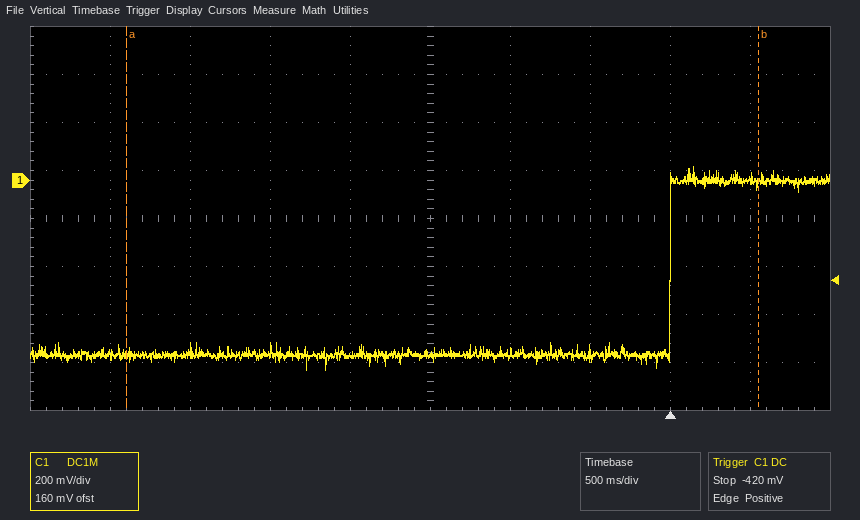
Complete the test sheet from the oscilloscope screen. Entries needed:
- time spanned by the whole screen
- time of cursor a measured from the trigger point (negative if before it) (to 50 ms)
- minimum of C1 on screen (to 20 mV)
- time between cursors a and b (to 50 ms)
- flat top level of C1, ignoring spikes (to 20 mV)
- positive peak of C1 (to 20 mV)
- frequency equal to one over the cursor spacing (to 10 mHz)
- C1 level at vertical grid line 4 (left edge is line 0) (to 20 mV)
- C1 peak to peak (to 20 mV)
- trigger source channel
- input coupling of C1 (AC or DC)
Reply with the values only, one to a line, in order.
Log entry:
5 s
-3.40 s
-780 mV
3.95 s
0 mV
60 mV
250 mHz
-720 mV
840 mV
C1
DC
